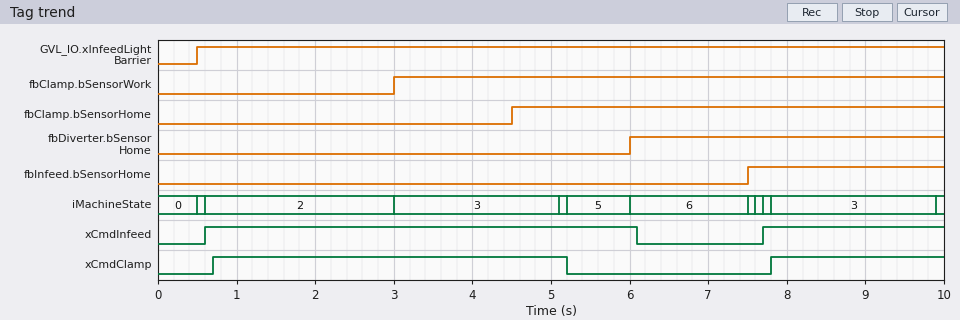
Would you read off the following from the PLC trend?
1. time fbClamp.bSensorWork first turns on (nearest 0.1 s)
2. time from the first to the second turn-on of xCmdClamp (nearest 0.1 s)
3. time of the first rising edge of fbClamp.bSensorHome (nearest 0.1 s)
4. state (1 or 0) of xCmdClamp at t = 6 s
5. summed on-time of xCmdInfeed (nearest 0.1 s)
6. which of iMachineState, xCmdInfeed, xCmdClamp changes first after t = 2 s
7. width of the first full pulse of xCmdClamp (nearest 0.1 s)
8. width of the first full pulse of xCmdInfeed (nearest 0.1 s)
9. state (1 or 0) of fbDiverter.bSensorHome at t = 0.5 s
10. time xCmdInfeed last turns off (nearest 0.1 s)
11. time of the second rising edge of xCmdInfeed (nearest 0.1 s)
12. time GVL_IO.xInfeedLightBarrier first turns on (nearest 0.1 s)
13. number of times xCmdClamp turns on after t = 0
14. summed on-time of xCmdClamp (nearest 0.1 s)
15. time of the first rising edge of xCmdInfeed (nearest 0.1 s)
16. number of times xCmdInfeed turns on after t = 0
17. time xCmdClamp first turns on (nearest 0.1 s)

3.0 s
7.1 s
4.5 s
0
7.8 s
iMachineState
4.5 s
5.5 s
0
6.1 s
7.7 s
0.5 s
2
6.7 s
0.6 s
2
0.7 s
